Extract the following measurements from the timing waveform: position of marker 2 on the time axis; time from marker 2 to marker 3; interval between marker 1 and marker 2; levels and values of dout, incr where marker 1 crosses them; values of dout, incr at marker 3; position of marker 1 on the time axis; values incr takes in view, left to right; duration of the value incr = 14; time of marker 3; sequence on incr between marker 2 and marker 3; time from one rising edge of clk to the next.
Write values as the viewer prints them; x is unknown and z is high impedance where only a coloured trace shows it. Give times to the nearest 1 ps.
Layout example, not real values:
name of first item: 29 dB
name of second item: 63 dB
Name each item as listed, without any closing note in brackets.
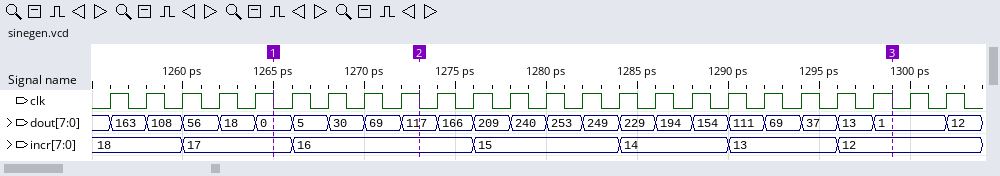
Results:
position of marker 2 on the time axis: 1273 ps
time from marker 2 to marker 3: 26 ps
interval between marker 1 and marker 2: 8 ps
levels and values of dout, incr where marker 1 crosses them: dout=0, incr=17
values of dout, incr at marker 3: dout=1, incr=12
position of marker 1 on the time axis: 1265 ps
values incr takes in view, left to right: 18, 17, 16, 15, 14, 13, 12
duration of the value incr = 14: 6 ps
time of marker 3: 1299 ps
sequence on incr between marker 2 and marker 3: 16, 15, 14, 13, 12
time from one rising edge of clk to the next: 2 ps
